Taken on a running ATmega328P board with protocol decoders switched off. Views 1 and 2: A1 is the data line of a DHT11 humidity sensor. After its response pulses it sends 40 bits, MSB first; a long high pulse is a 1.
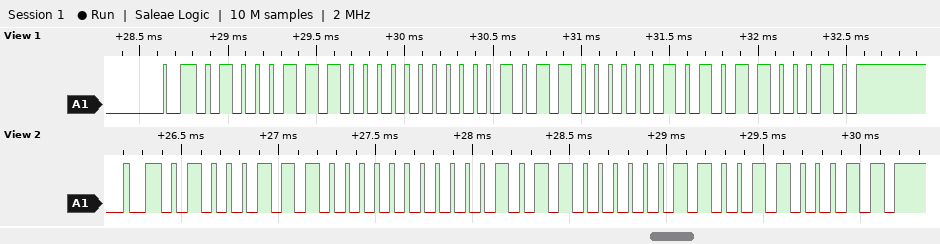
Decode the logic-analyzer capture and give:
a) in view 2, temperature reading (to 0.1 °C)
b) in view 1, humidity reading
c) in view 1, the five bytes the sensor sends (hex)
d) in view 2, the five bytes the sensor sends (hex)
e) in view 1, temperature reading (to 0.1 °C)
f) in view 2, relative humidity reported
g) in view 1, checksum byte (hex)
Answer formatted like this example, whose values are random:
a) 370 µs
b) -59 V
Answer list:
a) 22.6 °C
b) 71 %
c) 47 00 16 05 62
d) 47 00 16 06 63
e) 22.5 °C
f) 71 %
g) 0x62
